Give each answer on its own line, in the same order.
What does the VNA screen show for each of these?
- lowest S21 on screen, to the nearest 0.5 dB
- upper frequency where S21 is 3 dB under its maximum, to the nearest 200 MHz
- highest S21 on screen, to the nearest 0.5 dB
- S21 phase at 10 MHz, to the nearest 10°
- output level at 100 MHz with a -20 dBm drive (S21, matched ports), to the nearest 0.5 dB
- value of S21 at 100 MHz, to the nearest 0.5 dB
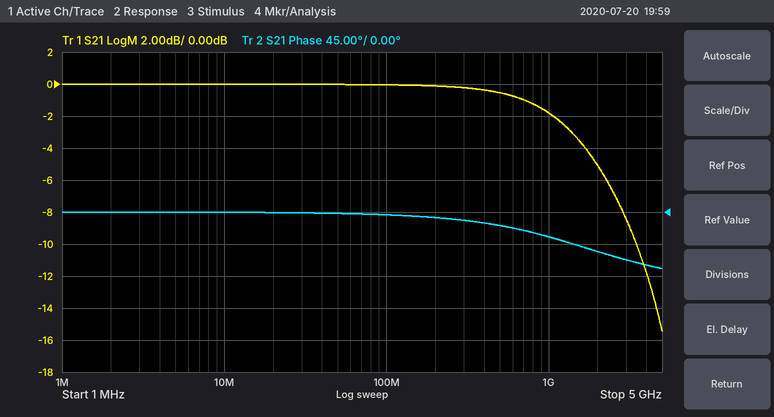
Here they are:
-15.5 dB
1.4 GHz
0.0 dB
0°
-20.0 dBm
0.0 dB
